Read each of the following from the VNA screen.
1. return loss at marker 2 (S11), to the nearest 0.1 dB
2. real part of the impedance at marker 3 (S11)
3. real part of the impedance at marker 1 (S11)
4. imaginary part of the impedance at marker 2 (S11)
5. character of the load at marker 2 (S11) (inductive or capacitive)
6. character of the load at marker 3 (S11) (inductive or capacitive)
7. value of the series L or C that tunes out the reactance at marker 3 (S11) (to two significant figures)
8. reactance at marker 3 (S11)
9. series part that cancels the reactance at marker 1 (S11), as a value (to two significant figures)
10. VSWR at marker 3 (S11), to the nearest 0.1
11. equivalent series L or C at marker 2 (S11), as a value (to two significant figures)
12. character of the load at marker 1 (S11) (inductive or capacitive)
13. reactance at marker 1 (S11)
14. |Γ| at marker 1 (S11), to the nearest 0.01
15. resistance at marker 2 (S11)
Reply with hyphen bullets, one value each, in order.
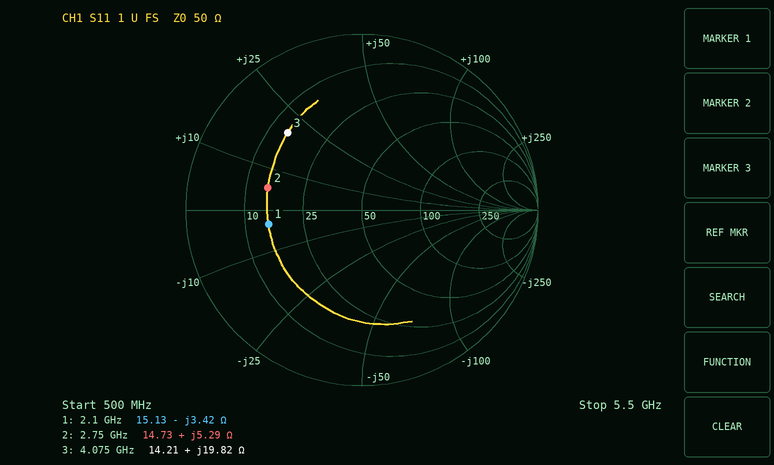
- 5.2 dB
- 14.21 Ω
- 15.13 Ω
- +5.29 Ω
- inductive
- inductive
- 2.0 pF
- +19.82 Ω
- 260 pH
- 4.1
- 310 pH
- capacitive
- -3.42 Ω
- 0.54
- 14.73 Ω
